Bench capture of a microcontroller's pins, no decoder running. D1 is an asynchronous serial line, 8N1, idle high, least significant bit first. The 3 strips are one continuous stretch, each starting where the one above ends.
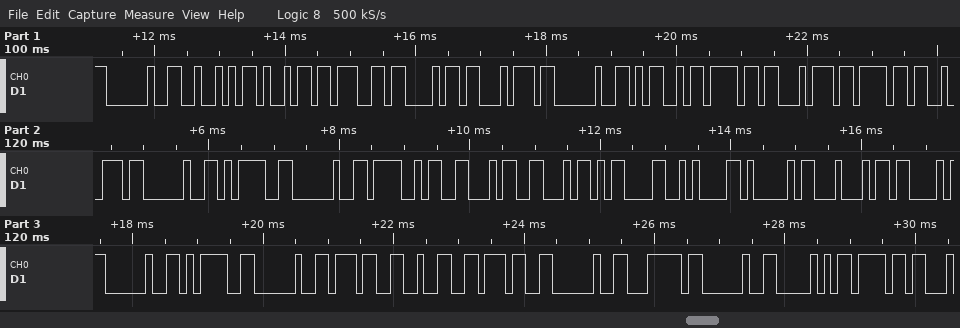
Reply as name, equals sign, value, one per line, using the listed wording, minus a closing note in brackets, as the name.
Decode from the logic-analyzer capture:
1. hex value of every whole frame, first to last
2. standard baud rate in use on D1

hex value of every whole frame, first to last = 0x20 0x52 0x69 0x67 0x68 0x74 0x20 0x4D 0x6F 0x74 0x6F 0x72 0x20 0x3D 0x20 0x4F 0x46 0x46 0x0D 0x0A 0x41 0x44 0x43 0x20 0x3D 0x20 0x37 0x32 0x37 0x20 0x7C 0x20 0x50 0x6F
standard baud rate in use on D1 = 9600 baud
